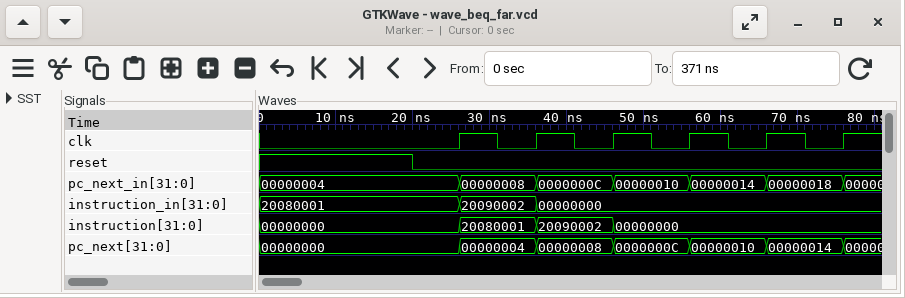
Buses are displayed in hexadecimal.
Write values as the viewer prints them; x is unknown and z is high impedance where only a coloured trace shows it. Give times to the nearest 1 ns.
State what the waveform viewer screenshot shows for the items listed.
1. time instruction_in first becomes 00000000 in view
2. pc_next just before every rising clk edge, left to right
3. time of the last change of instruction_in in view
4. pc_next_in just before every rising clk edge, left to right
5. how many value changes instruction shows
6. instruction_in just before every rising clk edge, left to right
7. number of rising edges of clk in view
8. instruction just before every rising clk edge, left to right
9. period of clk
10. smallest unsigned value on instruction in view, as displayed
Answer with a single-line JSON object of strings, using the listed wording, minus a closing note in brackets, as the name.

{"time instruction_in first becomes 00000000 in view": "36 ns", "pc_next just before every rising clk edge, left to right": "00000000, 00000004, 00000008, 0000000C, 00000010, 00000014", "time of the last change of instruction_in in view": "36 ns", "pc_next_in just before every rising clk edge, left to right": "00000004, 00000008, 0000000C, 00000010, 00000014, 00000018", "how many value changes instruction shows": "3", "instruction_in just before every rising clk edge, left to right": "20080001, 20090002, 00000000, 00000000, 00000000, 00000000", "number of rising edges of clk in view": "6", "instruction just before every rising clk edge, left to right": "00000000, 20080001, 20090002, 00000000, 00000000, 00000000", "period of clk": "10 ns", "smallest unsigned value on instruction in view, as displayed": "00000000"}
